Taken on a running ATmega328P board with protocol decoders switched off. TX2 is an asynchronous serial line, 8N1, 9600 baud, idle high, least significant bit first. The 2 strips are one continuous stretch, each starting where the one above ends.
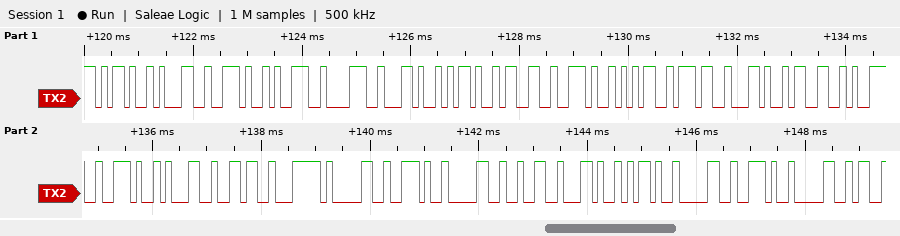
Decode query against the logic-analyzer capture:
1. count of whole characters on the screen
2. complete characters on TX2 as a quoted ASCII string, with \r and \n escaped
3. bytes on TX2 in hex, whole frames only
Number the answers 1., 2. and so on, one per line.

1. 27
2. "-1.98,-3.57,39.16|0.02,-0.0"
3. 2D 31 2E 39 38 2C 2D 33 2E 35 37 2C 33 39 2E 31 36 7C 30 2E 30 32 2C 2D 30 2E 30
